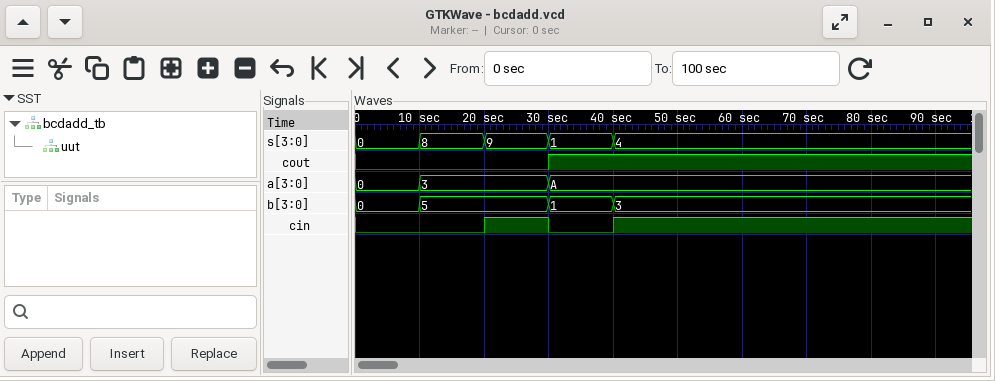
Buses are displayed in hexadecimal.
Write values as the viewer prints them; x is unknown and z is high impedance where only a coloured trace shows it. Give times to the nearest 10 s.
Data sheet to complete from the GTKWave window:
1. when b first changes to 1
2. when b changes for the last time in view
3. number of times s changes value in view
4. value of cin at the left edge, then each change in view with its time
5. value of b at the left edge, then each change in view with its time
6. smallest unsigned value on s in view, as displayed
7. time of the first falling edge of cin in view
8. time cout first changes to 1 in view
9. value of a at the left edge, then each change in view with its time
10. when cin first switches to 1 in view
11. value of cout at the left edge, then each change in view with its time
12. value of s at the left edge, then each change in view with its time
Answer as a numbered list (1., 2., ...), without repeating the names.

1. 30 s
2. 40 s
3. 4
4. 0, 1 at 20 s, 0 at 30 s, 1 at 40 s
5. 0, 5 at 10 s, 1 at 30 s, 3 at 40 s
6. 0
7. 30 s
8. 30 s
9. 0, 3 at 10 s, A at 30 s
10. 20 s
11. 0, 1 at 30 s
12. 0, 8 at 10 s, 9 at 20 s, 1 at 30 s, 4 at 40 s
